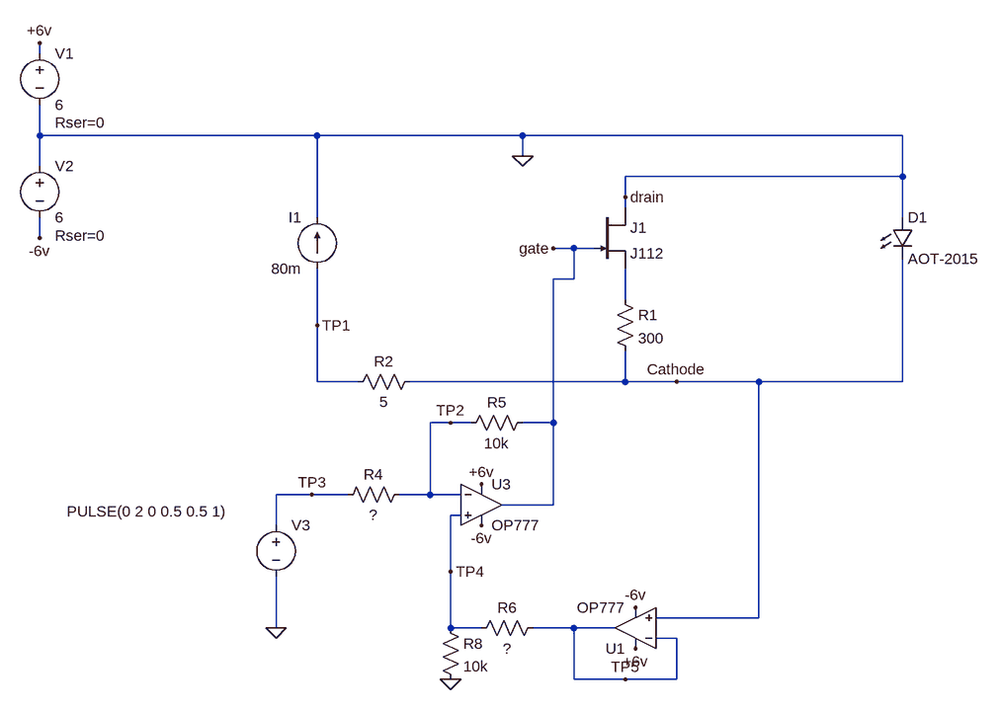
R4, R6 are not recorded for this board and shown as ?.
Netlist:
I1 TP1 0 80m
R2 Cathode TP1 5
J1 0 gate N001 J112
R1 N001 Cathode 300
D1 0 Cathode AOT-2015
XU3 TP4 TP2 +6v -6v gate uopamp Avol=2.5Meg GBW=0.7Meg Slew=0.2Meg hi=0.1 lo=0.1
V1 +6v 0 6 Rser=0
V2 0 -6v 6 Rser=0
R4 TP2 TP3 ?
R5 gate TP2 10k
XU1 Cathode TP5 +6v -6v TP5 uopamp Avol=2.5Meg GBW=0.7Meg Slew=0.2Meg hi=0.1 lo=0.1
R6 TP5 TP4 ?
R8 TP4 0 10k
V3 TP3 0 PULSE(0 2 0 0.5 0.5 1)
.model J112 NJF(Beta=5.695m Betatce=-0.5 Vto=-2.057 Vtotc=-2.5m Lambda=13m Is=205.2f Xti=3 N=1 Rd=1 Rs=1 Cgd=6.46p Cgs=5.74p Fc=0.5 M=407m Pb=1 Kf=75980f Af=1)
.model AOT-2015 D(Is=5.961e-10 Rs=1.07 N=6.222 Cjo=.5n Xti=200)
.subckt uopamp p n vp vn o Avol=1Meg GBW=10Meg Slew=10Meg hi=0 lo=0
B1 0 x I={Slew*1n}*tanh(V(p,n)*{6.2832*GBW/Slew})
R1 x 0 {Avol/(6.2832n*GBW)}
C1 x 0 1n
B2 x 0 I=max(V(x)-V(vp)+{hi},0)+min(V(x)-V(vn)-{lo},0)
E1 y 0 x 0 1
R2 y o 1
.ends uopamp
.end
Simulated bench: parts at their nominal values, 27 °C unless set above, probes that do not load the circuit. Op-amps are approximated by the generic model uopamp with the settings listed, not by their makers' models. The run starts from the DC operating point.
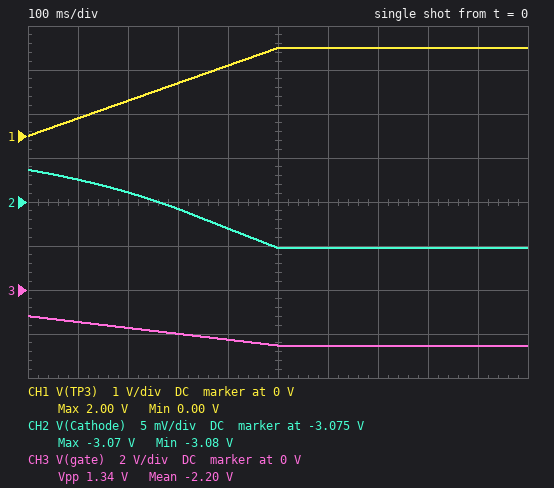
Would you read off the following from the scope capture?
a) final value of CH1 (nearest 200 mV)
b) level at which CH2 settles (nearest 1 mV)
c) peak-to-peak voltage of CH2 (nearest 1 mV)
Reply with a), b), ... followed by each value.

a) 2.0 V
b) -3.080 V
c) 9 mV
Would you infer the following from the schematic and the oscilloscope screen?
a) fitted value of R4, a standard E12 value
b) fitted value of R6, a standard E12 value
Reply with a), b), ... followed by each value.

a) 15 kΩ
b) 33 kΩ
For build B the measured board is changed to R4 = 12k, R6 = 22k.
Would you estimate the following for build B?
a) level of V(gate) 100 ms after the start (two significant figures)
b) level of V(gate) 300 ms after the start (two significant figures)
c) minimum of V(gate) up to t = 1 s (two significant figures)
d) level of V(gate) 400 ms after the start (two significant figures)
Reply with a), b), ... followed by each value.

a) -2.1 V
b) -2.8 V
c) -3.4 V
d) -3.1 V
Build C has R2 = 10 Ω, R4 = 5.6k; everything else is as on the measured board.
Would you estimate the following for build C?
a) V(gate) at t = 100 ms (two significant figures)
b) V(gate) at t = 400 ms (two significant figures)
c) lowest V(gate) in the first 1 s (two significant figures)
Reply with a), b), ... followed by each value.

a) -2.7 V
b) -4.9 V
c) -5.6 V
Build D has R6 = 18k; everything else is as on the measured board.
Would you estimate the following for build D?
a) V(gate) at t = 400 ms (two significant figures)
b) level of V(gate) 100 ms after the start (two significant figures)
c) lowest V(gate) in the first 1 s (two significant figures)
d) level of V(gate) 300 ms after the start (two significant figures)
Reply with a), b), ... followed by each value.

a) -2.9 V
b) -2.1 V
c) -3.2 V
d) -2.6 V
